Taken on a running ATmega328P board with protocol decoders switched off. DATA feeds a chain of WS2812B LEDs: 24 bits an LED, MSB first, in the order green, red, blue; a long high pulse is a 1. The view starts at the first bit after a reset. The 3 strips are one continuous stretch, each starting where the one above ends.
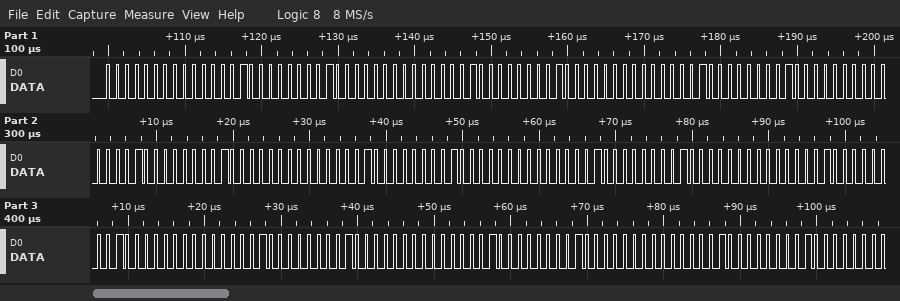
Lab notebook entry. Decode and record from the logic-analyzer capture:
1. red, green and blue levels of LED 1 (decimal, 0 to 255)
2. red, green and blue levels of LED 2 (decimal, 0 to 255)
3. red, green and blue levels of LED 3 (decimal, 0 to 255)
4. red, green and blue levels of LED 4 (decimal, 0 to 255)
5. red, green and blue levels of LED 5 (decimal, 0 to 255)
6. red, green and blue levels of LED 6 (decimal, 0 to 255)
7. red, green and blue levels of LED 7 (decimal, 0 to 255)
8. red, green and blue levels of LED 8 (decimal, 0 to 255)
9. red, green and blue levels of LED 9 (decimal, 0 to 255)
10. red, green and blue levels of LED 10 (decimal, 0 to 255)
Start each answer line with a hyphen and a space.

- 2, 0, 1
- 2, 0, 1
- 2, 0, 1
- 2, 0, 1
- 2, 0, 1
- 2, 0, 1
- 2, 0, 1
- 2, 0, 1
- 2, 0, 1
- 2, 0, 1
